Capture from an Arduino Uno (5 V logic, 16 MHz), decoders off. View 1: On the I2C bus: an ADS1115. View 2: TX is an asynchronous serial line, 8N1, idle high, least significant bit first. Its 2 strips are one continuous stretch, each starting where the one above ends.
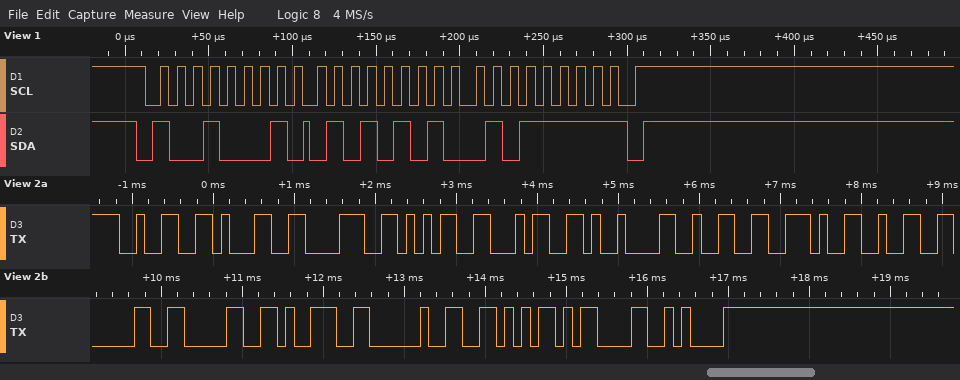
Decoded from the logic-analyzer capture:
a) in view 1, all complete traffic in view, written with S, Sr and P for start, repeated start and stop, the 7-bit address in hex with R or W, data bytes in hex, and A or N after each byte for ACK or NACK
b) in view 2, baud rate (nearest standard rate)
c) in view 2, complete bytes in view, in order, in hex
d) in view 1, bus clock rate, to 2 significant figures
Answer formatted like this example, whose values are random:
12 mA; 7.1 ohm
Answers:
S 48R A 55 A 5F N P; 9600 baud; 0x32 0x31 0x38 0x35 0x34 0x09 0x32 0x2E 0x32 0x30 0x30 0x39 0x20 0x56 0x0D 0x0A; 100 kHz
